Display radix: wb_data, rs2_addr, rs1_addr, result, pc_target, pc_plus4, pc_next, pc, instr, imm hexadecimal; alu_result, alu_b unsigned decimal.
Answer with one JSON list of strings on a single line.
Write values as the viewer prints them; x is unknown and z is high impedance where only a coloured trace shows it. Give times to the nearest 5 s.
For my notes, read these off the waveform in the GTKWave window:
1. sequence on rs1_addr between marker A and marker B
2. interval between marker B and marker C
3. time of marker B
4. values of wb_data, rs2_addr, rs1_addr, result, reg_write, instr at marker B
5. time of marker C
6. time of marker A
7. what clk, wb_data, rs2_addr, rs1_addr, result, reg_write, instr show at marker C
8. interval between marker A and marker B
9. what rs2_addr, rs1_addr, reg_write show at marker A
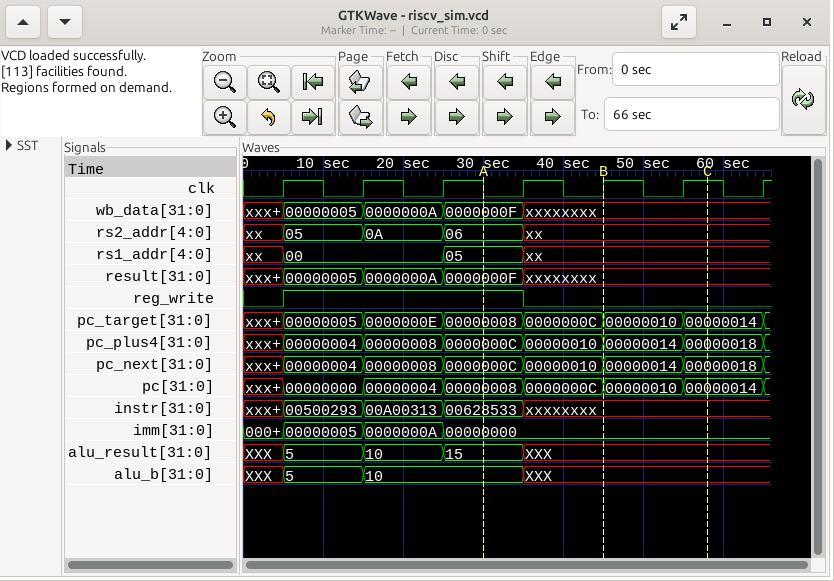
["05, xx", "15 s", "45 s", "wb_data=xxxxxxxx, rs2_addr=xx, rs1_addr=xx, result=xxxxxxxx, reg_write=0, instr=xxxxxxxx", "60 s", "30 s", "clk=1, wb_data=xxxxxxxx, rs2_addr=xx, rs1_addr=xx, result=xxxxxxxx, reg_write=0, instr=xxxxxxxx", "15 s", "rs2_addr=06, rs1_addr=05, reg_write=1"]
